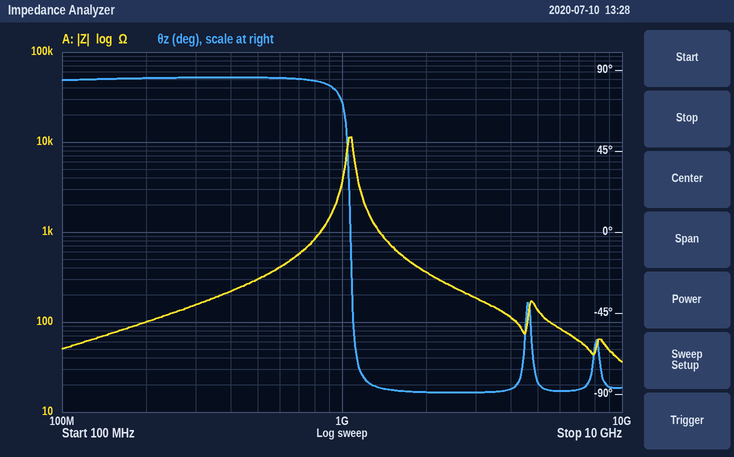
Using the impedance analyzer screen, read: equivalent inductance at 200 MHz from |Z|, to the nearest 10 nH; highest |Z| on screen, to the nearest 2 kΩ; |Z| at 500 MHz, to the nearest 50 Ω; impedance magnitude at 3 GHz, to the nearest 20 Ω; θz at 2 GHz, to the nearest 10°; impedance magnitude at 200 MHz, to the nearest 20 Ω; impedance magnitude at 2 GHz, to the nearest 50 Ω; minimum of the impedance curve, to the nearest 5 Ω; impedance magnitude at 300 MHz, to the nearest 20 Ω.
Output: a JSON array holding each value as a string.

["80 nH", "12 kΩ", "300 Ω", "180 Ω", "-90°", "100 Ω", "350 Ω", "35 Ω", "160 Ω"]
